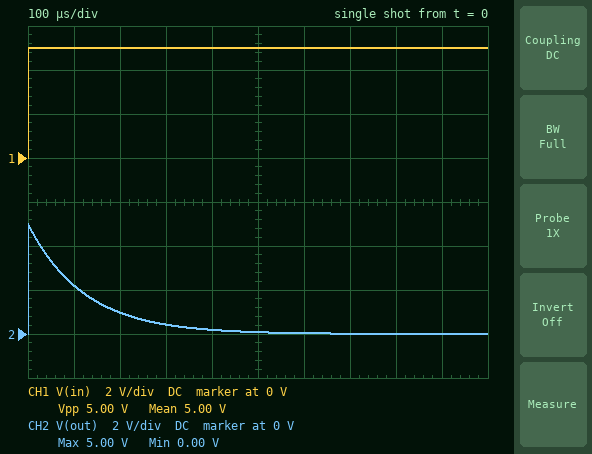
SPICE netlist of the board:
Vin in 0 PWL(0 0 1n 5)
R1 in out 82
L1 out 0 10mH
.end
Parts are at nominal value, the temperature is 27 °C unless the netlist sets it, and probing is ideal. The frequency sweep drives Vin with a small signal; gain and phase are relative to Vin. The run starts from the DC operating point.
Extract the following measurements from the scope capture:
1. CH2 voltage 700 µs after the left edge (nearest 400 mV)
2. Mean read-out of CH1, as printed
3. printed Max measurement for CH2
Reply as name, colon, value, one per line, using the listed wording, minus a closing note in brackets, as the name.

CH2 voltage 700 µs after the left edge: 0 V
Mean read-out of CH1, as printed: 5.00 V
printed Max measurement for CH2: 5.00 V
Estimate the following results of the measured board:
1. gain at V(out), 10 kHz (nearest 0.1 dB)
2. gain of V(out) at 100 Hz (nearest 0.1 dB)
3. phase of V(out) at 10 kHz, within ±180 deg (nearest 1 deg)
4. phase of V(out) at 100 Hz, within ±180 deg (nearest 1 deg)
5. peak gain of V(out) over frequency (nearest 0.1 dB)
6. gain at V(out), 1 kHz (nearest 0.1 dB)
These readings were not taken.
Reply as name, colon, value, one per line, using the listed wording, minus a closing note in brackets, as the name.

gain at V(out), 10 kHz: -0.1 dB
gain of V(out) at 100 Hz: -22.3 dB
phase of V(out) at 10 kHz, within ±180 deg: 7 deg
phase of V(out) at 100 Hz, within ±180 deg: 86 deg
peak gain of V(out) over frequency: 0 dB
gain at V(out), 1 kHz: -4.3 dB
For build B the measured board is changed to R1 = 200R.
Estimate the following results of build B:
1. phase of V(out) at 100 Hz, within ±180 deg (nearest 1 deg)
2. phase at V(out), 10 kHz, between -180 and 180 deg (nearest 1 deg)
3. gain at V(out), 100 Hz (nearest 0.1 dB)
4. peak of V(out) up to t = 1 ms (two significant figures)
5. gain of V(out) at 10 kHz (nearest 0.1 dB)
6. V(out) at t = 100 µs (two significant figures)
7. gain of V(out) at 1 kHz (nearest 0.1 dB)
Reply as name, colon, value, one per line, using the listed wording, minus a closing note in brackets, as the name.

phase of V(out) at 100 Hz, within ±180 deg: 88 deg
phase at V(out), 10 kHz, between -180 and 180 deg: 18 deg
gain at V(out), 100 Hz: -30.1 dB
peak of V(out) up to t = 1 ms: 5.0 V
gain of V(out) at 10 kHz: -0.4 dB
V(out) at t = 100 µs: 680 mV
gain of V(out) at 1 kHz: -10.5 dB
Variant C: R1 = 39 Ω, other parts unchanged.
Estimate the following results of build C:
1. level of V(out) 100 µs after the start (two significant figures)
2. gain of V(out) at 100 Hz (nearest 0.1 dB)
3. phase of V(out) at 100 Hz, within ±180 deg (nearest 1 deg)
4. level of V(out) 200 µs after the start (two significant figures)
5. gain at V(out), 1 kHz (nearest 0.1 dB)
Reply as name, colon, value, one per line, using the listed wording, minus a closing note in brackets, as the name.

level of V(out) 100 µs after the start: 3.4 V
gain of V(out) at 100 Hz: -16.0 dB
phase of V(out) at 100 Hz, within ±180 deg: 81 deg
level of V(out) 200 µs after the start: 2.3 V
gain at V(out), 1 kHz: -1.4 dB
